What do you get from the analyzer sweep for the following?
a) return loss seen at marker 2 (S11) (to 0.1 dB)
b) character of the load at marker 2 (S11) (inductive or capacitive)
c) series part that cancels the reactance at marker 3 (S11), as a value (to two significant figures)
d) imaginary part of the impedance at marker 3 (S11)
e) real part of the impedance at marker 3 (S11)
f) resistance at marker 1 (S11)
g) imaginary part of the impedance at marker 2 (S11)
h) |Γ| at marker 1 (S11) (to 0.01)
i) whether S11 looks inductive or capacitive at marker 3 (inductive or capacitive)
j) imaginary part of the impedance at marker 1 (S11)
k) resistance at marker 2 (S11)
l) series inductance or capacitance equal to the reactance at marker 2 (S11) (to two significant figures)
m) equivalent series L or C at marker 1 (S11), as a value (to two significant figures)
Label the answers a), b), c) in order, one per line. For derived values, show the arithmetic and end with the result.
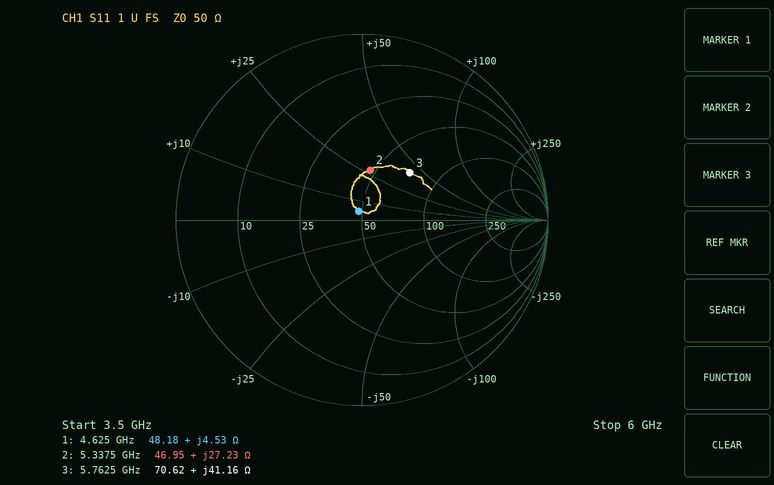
a) 11.3 dB
b) inductive
c) C = 1/(2π × 5.7625 GHz × 41.16 Ω) ≈ 671 fF, so 670 fF to two significant figures
d) +41.16 Ω
e) 70.62 Ω
f) 48.18 Ω
g) +27.23 Ω
h) 0.05
i) inductive
j) +4.53 Ω
k) 46.95 Ω
l) L = 27.23 Ω/(2π × 5.3375 GHz) ≈ 812 pH, so 810 pH to two significant figures
m) L = 4.53 Ω/(2π × 4.625 GHz) ≈ 156 pH, so 160 pH to two significant figures
